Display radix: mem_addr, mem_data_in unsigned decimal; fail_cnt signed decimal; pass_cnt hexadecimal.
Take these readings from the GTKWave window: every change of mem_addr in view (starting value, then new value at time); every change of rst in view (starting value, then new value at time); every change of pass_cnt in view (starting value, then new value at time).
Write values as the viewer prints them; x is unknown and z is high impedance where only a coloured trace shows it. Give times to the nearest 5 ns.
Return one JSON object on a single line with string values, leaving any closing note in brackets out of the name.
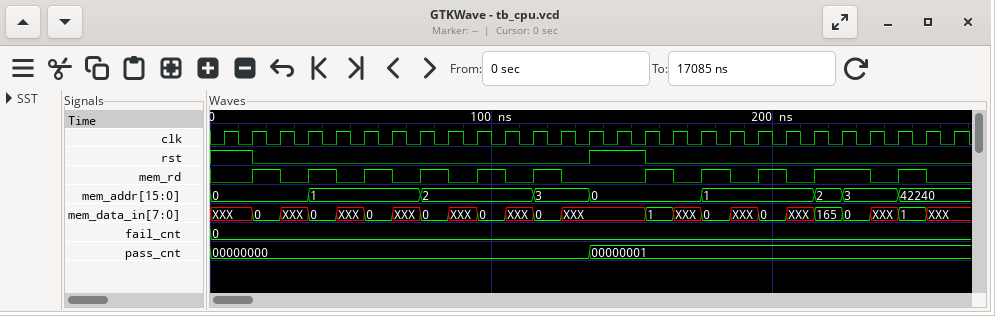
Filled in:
{"every change of mem_addr in view": "0, 1 at 35 ns, 2 at 75 ns, 3 at 115 ns, 0 at 135 ns, 1 at 175 ns, 2 at 215 ns, 3 at 225 ns, 42240 at 245 ns", "every change of rst in view": "1, 0 at 15 ns, 1 at 135 ns, 0 at 155 ns", "every change of pass_cnt in view": "00000000, 00000001 at 135 ns"}
